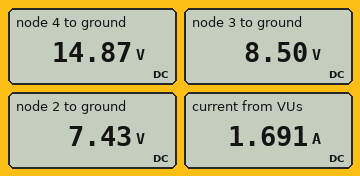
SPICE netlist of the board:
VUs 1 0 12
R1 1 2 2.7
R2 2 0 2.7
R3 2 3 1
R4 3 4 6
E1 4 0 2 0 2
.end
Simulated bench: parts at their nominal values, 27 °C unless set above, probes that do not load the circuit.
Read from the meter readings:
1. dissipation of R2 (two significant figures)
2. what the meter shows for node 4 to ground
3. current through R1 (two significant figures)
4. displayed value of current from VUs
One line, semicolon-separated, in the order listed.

20 W; 14.87 V; 1.7 A; 1.691 A
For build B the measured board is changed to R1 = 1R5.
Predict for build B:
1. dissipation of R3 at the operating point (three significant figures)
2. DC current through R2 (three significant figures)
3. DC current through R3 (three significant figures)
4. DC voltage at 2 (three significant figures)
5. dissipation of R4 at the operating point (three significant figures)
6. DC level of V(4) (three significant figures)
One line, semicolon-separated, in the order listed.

1.63 W; 3.31 A; 1.28 A; 8.95 V; 9.80 W; 17.9 V
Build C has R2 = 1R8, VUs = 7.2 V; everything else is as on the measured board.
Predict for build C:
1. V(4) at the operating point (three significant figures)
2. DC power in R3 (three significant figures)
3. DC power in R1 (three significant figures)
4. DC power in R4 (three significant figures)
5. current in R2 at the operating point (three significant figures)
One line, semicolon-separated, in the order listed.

6.81 V; 237 mW; 5.33 W; 1.42 W; 1.89 A
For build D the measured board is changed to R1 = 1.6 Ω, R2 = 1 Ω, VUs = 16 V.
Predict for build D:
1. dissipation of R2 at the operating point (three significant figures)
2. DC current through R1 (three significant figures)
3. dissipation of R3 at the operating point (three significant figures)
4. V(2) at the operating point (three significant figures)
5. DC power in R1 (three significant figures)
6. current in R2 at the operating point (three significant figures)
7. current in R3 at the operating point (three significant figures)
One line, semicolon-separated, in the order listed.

45.5 W; 5.78 A; 929 mW; 6.75 V; 53.5 W; 6.75 A; 964 mA
